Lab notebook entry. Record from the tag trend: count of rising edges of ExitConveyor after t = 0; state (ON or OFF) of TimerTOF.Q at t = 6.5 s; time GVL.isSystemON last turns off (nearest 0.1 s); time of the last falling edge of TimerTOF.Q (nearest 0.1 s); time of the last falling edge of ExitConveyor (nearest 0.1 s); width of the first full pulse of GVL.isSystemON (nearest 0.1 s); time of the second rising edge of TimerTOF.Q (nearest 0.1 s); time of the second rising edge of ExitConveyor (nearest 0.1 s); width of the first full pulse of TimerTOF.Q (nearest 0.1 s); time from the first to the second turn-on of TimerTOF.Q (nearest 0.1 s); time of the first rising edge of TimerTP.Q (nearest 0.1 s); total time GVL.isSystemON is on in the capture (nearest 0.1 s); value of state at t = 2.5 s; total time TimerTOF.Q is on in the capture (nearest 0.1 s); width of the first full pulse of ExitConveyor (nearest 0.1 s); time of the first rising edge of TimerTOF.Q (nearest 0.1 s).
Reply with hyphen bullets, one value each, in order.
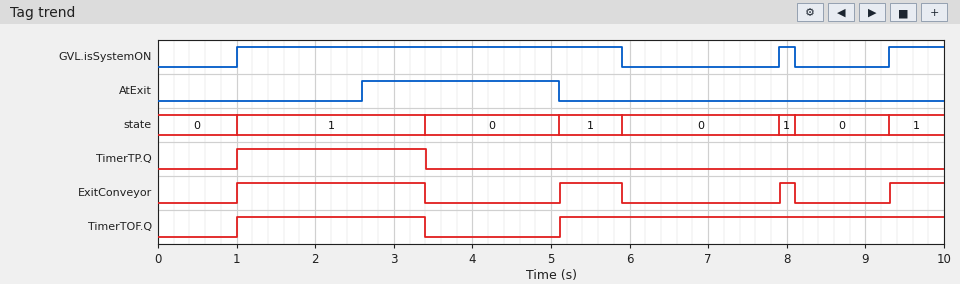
- 4
- ON
- 8.1 s
- 3.4 s
- 8.1 s
- 4.9 s
- 5.1 s
- 5.1 s
- 2.4 s
- 4.1 s
- 1.0 s
- 5.8 s
- 1
- 7.3 s
- 2.4 s
- 1.0 s
